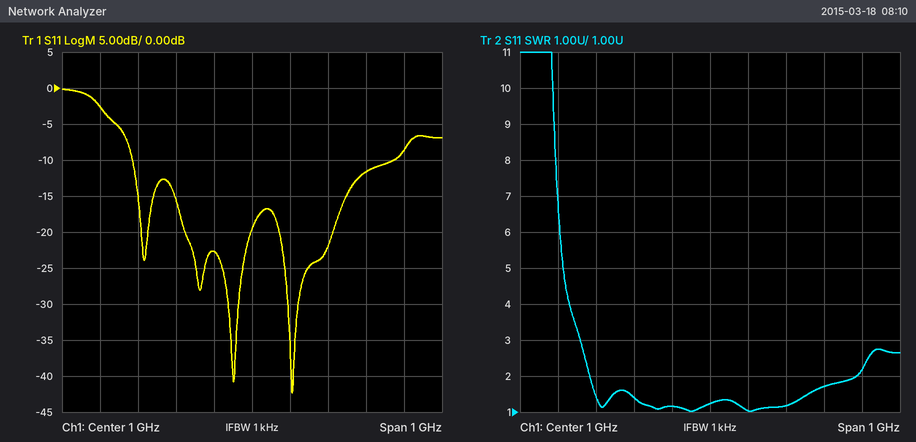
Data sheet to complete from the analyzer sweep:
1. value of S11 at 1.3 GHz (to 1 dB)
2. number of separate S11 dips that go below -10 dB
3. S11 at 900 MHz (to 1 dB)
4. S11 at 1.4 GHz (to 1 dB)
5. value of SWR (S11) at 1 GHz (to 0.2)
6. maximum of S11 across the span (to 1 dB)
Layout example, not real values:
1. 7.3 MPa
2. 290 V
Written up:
1. -12 dB
2. 4
3. -23 dB
4. -9 dB
5. 1.2
6. 0 dB
